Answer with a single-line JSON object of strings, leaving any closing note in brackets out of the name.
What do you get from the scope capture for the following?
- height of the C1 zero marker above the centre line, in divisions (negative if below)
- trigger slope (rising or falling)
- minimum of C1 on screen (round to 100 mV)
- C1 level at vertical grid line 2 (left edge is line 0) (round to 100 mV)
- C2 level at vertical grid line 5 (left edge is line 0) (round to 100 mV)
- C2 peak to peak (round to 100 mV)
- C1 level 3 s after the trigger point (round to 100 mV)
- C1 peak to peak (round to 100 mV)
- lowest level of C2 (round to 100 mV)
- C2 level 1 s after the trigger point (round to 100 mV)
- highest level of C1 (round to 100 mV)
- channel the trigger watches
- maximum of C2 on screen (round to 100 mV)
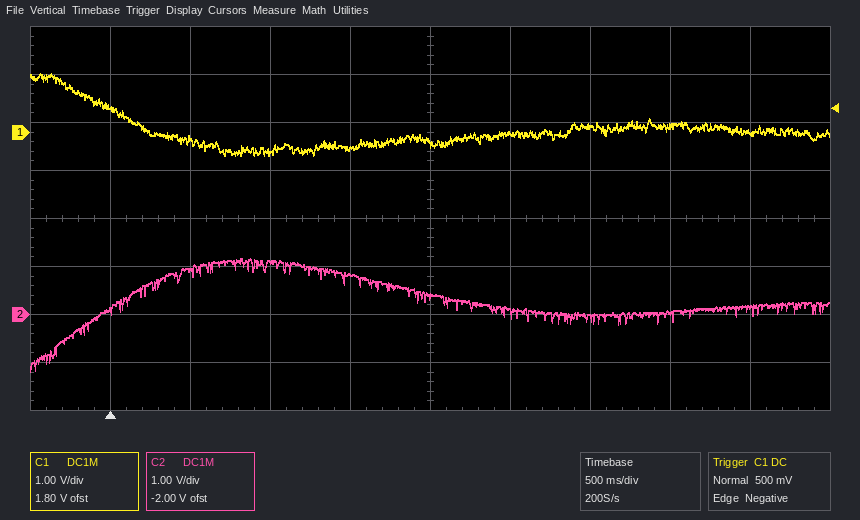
{"height of the C1 zero marker above the centre line, in divisions": "+1.8 div", "trigger slope": "falling", "minimum of C1 on screen": "-500 mV", "C1 level at vertical grid line 2 (left edge is line 0)": "-200 mV", "C2 level at vertical grid line 5 (left edge is line 0)": "400 mV", "C2 peak to peak": "2.4 V", "C1 level 3 s after the trigger point": "100 mV", "C1 peak to peak": "1.7 V", "lowest level of C2": "-1.2 V", "C2 level 1 s after the trigger point": "1.1 V", "highest level of C1": "1.2 V", "channel the trigger watches": "C1", "maximum of C2 on screen": "1.2 V"}
